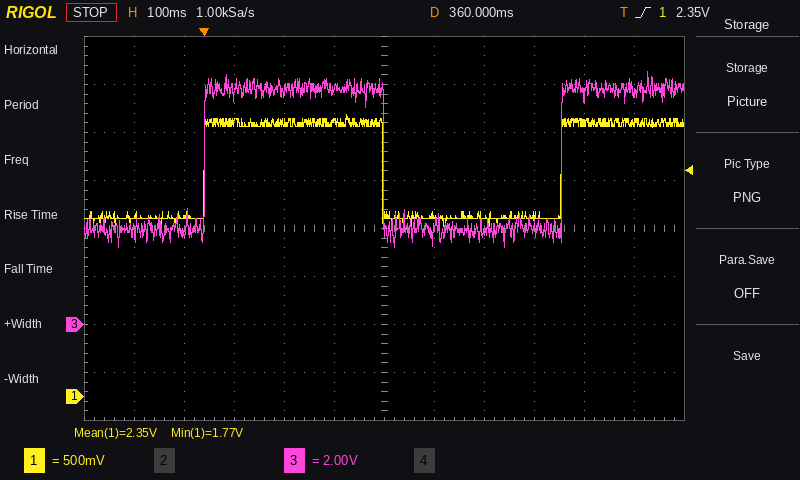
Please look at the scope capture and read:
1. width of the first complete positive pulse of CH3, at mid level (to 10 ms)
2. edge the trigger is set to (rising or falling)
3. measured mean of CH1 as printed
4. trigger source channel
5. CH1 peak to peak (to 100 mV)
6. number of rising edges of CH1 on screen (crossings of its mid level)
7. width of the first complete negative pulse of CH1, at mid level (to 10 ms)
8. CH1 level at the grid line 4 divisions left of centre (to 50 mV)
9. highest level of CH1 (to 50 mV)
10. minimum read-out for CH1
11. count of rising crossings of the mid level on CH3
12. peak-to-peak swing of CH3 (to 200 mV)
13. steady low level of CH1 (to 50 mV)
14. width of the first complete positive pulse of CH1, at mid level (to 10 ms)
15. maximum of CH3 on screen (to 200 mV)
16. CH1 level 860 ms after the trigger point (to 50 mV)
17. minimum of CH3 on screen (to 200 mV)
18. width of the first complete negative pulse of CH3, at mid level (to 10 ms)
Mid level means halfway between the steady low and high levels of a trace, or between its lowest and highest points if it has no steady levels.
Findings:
360 ms
rising
2.35 V
CH1
1.20 V
2
360 ms
1.90 V
2.95 V
1.77 V
2
7.4 V
1.85 V
360 ms
10.6 V
2.85 V
3.2 V
360 ms
